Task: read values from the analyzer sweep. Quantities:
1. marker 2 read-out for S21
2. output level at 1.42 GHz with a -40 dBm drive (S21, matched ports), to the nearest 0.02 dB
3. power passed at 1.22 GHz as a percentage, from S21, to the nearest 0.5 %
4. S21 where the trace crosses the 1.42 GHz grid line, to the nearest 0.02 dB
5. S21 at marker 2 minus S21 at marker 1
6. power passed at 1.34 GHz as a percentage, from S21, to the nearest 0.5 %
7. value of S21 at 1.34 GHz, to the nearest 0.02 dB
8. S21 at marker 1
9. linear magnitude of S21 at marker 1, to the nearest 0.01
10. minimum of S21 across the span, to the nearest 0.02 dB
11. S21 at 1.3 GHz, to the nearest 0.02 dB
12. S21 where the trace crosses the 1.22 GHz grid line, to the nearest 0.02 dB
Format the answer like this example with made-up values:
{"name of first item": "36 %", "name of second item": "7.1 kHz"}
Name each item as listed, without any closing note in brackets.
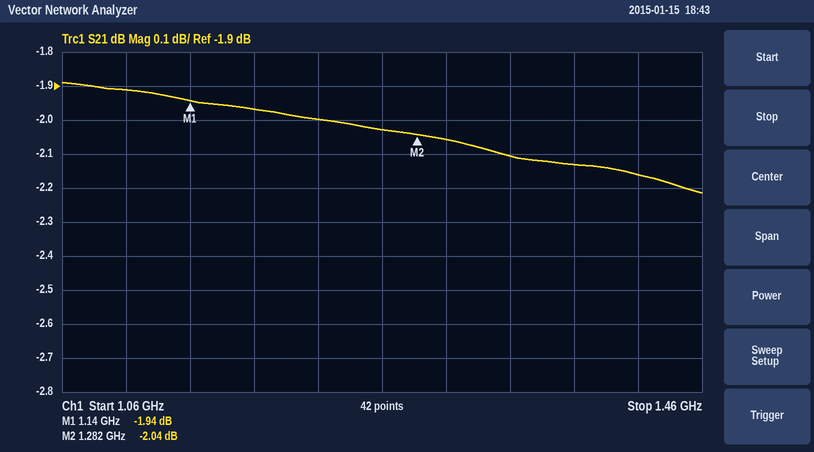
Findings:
{"marker 2 read-out for S21": "-2.04 dB", "output level at 1.42 GHz with a -40 dBm drive (S21, matched ports), to the nearest 0.02 dB": "-42.16 dBm", "power passed at 1.22 GHz as a percentage, from S21, to the nearest 0.5 %": "63.0 %", "S21 where the trace crosses the 1.42 GHz grid line, to the nearest 0.02 dB": "-2.16 dB", "S21 at marker 2 minus S21 at marker 1": "-0.10 dB", "power passed at 1.34 GHz as a percentage, from S21, to the nearest 0.5 %": "61.5 %", "value of S21 at 1.34 GHz, to the nearest 0.02 dB": "-2.10 dB", "S21 at marker 1": "-1.94 dB", "linear magnitude of S21 at marker 1, to the nearest 0.01": "0.80", "minimum of S21 across the span, to the nearest 0.02 dB": "-2.22 dB", "S21 at 1.3 GHz, to the nearest 0.02 dB": "-2.06 dB", "S21 where the trace crosses the 1.22 GHz grid line, to the nearest 0.02 dB": "-2.00 dB"}
